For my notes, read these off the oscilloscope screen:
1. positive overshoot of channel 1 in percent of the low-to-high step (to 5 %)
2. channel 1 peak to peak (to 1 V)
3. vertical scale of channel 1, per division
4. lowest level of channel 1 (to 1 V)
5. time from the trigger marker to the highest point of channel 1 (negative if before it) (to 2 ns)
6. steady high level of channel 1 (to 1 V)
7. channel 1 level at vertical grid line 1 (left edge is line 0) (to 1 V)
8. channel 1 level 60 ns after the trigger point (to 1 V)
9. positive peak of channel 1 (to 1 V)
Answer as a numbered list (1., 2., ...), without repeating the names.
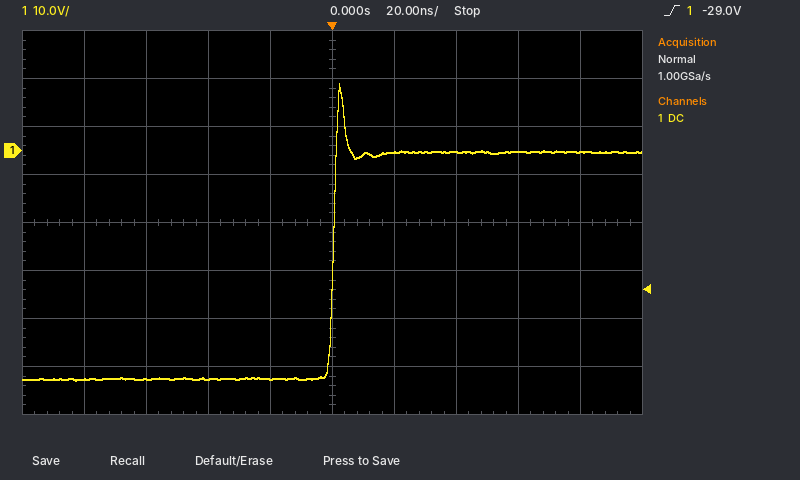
1. 30 %
2. 62 V
3. 10 V
4. -48 V
5. +2 ns
6. 0 V
7. -48 V
8. 0 V
9. 14 V
